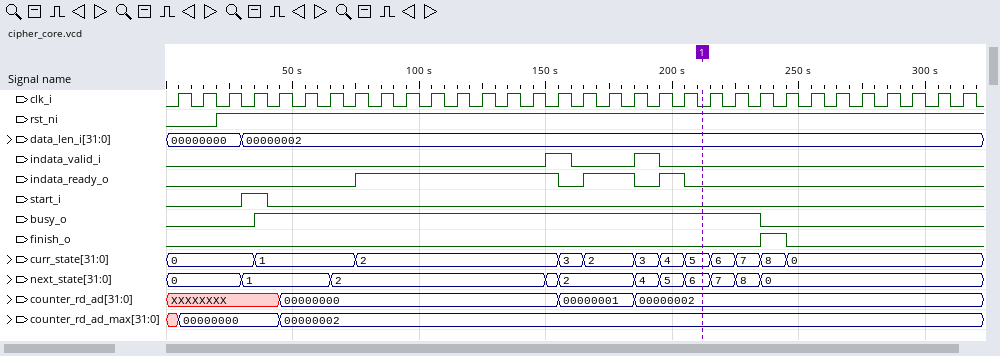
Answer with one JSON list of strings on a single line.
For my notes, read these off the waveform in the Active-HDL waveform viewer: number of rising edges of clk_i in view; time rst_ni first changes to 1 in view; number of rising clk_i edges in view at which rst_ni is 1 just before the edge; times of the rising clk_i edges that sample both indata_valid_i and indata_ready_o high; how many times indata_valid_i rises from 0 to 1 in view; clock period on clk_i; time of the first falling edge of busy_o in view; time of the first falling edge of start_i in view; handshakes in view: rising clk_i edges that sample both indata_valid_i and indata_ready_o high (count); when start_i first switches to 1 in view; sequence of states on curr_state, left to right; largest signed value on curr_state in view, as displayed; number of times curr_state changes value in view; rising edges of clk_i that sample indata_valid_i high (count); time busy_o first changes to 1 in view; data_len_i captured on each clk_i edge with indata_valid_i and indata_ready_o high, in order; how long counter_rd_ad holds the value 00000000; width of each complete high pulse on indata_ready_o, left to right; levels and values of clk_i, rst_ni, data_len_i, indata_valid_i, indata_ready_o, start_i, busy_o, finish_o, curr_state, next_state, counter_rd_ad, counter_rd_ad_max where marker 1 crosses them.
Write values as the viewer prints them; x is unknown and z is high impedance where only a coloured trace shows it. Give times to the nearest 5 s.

["32", "20 s", "30", "155 s", "2", "10 s", "235 s", "40 s", "1", "30 s", "0, 1, 2, 3, 2, 3, 4, 5, 6, 7, 8, 0", "8", "11", "2", "35 s", "00000002", "110 s", "80 s, 20 s, 10 s", "clk_i=0, rst_ni=1, data_len_i=00000002, indata_valid_i=0, indata_ready_o=0, start_i=0, busy_o=1, finish_o=0, curr_state=5, next_state=6, counter_rd_ad=00000002, counter_rd_ad_max=00000002"]
